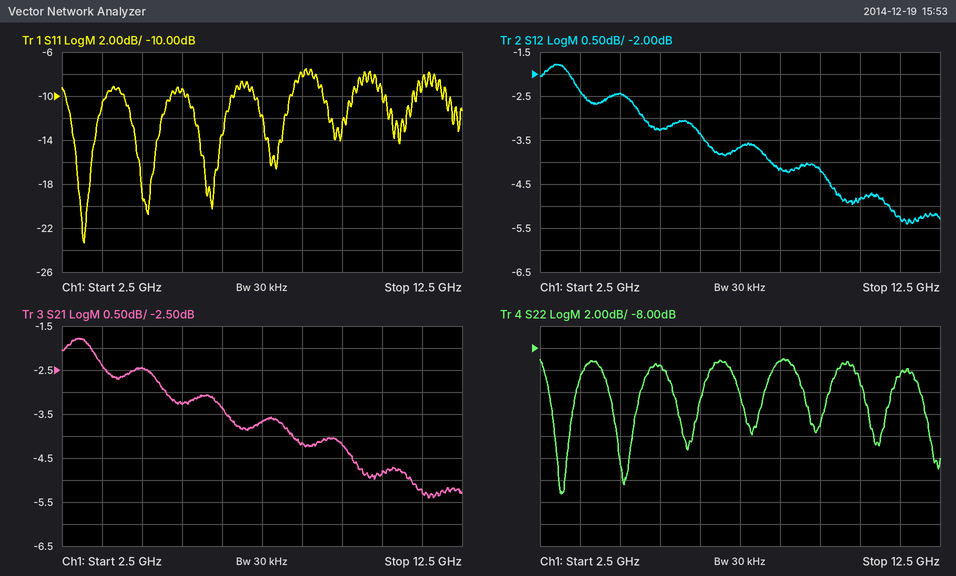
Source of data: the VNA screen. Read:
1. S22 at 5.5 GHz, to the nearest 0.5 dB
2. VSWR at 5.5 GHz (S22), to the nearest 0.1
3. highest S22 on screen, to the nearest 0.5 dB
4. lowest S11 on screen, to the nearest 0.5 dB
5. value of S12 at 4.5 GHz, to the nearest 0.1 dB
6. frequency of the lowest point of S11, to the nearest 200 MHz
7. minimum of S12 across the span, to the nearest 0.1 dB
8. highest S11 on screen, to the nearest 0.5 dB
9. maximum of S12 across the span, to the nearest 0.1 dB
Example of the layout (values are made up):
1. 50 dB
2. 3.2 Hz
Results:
1. -9.5 dB
2. 2.0
3. -9.0 dB
4. -23.5 dB
5. -2.4 dB
6. 3.0 GHz
7. -5.4 dB
8. -7.5 dB
9. -1.8 dB
